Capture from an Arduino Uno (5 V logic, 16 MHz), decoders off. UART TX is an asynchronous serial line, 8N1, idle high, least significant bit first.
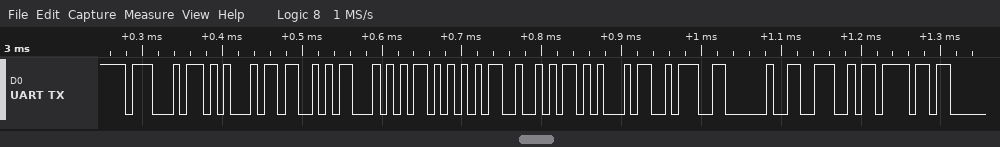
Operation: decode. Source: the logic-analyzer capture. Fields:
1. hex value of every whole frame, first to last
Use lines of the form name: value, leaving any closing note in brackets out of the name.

hex value of every whole frame, first to last: 0x47 0x45 0x53 0x54 0x55 0x52 0x45 0x3A 0x20 0x4E 0x6F
